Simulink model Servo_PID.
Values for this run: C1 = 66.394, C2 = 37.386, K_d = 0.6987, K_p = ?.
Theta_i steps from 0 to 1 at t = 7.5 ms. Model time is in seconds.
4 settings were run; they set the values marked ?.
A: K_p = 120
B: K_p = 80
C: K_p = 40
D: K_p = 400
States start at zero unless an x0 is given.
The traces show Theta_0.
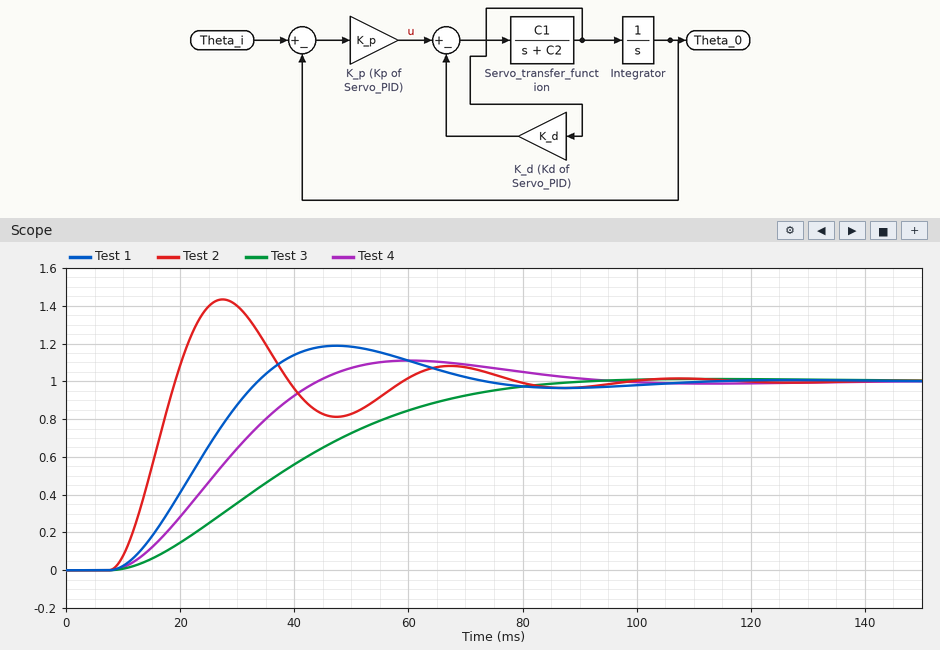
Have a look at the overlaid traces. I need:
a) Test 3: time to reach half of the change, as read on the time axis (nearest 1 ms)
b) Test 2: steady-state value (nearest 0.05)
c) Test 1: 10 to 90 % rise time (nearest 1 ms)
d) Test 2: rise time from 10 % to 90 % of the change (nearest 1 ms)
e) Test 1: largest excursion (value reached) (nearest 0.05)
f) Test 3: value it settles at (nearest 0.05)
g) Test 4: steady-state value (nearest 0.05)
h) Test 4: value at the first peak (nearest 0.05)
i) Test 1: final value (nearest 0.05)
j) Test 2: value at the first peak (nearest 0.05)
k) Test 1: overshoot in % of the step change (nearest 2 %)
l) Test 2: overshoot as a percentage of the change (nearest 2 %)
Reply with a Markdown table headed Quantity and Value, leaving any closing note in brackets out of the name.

| Quantity | Value |
|---|---|
| Test 3: time to reach half of the change, as read on the time axis | 37 ms |
| Test 2: steady-state value | 1.00 |
| Test 1: 10 to 90 % rise time | 18 ms |
| Test 2: rise time from 10 % to 90 % of the change | 8 ms |
| Test 1: largest excursion (value reached) | 1.20 |
| Test 3: value it settles at | 1.00 |
| Test 4: steady-state value | 1.00 |
| Test 4: value at the first peak | 1.10 |
| Test 1: final value | 1.00 |
| Test 2: value at the first peak | 1.45 |
| Test 1: overshoot in % of the step change | 18 % |
| Test 2: overshoot as a percentage of the change | 44 % |
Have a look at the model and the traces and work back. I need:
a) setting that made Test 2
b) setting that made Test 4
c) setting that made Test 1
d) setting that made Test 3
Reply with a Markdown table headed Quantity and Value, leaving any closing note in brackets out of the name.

| Quantity | Value |
|---|---|
| setting that made Test 2 | D |
| setting that made Test 4 | B |
| setting that made Test 1 | A |
| setting that made Test 3 | C |
